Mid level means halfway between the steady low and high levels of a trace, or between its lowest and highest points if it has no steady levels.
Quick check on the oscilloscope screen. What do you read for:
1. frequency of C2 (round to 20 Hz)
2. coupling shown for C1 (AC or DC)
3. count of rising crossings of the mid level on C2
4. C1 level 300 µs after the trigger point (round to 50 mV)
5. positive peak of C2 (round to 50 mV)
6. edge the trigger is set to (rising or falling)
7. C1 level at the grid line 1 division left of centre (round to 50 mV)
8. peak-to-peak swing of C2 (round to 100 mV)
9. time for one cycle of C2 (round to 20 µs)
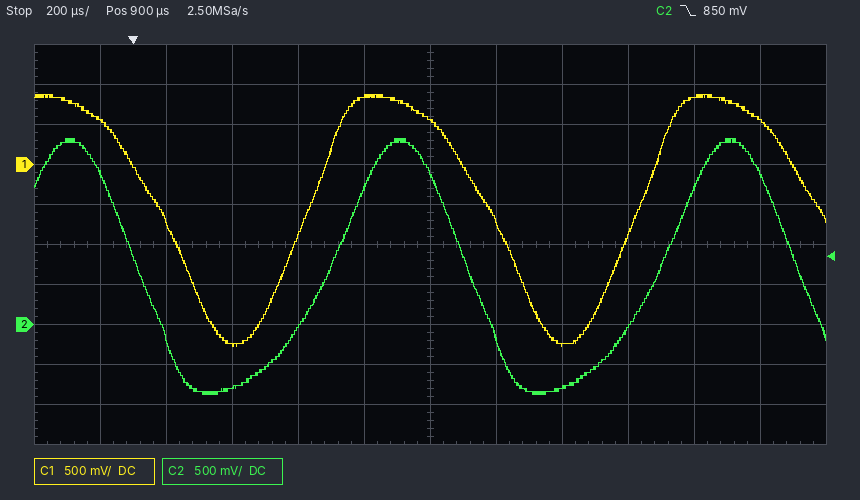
1.00 kHz
DC
2
-2.25 V
2.30 V
falling
850 mV
3.20 V
1.00 ms
